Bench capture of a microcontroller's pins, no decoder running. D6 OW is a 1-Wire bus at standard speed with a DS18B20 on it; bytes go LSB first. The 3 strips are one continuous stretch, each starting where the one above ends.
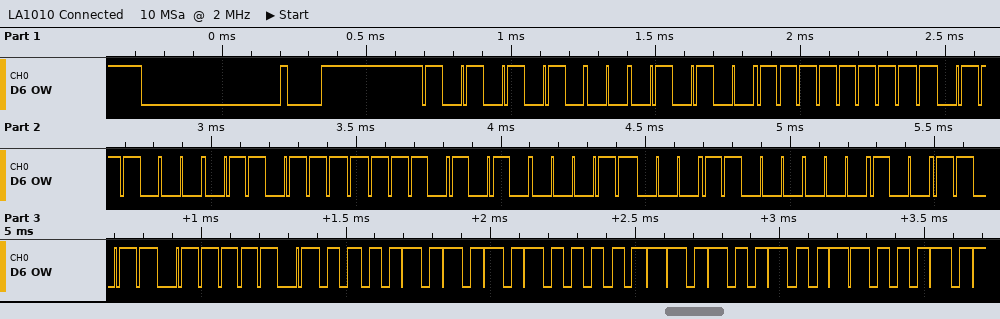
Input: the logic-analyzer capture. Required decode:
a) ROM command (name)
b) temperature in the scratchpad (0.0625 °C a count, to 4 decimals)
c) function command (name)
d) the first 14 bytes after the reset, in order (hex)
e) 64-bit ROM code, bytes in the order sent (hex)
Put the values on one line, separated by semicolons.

Match ROM; 85.0000 °C; Read Scratchpad; 55 28 FF 1D F6 57 18 03 D9 BE 50 05 4B 46; 28 FF 1D F6 57 18 03 D9
